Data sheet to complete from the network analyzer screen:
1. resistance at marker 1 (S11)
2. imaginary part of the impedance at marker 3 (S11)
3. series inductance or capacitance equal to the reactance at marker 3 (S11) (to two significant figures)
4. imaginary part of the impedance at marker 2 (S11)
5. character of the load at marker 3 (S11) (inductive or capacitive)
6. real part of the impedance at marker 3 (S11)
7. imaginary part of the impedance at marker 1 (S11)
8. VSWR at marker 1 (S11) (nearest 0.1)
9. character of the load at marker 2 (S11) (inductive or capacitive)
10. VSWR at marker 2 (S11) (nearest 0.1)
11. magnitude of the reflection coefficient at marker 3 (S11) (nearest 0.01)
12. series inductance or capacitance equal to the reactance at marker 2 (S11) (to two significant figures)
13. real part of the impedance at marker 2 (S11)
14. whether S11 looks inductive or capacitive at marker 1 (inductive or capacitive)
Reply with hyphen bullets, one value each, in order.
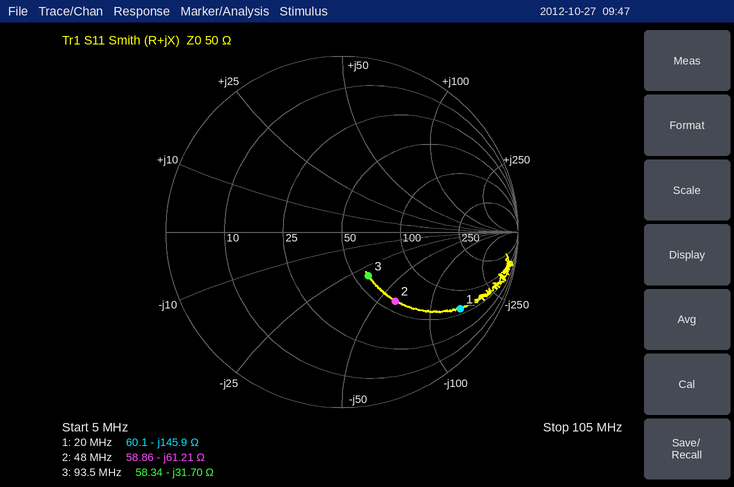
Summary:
- 60.1 Ω
- -31.70 Ω
- 54 pF
- -61.21 Ω
- capacitive
- 58.34 Ω
- -145.9 Ω
- 9.0
- capacitive
- 3.0
- 0.29
- 54 pF
- 58.86 Ω
- capacitive
